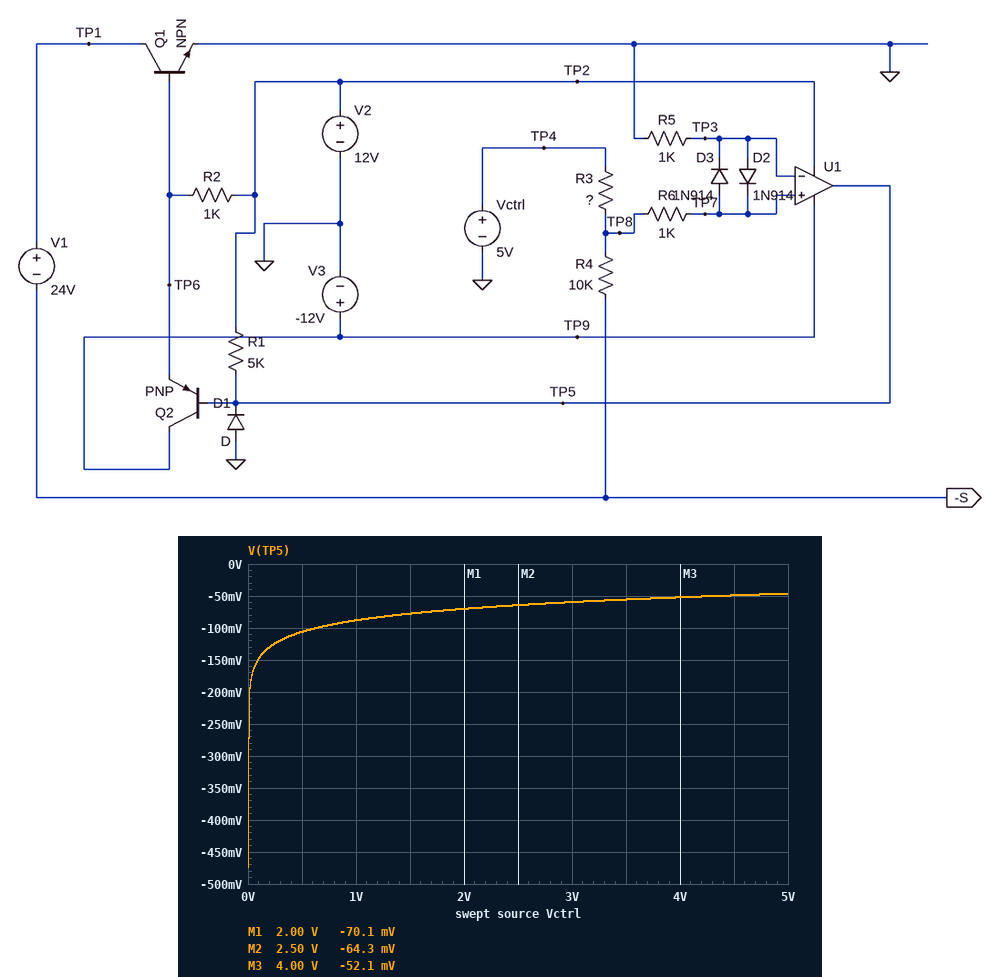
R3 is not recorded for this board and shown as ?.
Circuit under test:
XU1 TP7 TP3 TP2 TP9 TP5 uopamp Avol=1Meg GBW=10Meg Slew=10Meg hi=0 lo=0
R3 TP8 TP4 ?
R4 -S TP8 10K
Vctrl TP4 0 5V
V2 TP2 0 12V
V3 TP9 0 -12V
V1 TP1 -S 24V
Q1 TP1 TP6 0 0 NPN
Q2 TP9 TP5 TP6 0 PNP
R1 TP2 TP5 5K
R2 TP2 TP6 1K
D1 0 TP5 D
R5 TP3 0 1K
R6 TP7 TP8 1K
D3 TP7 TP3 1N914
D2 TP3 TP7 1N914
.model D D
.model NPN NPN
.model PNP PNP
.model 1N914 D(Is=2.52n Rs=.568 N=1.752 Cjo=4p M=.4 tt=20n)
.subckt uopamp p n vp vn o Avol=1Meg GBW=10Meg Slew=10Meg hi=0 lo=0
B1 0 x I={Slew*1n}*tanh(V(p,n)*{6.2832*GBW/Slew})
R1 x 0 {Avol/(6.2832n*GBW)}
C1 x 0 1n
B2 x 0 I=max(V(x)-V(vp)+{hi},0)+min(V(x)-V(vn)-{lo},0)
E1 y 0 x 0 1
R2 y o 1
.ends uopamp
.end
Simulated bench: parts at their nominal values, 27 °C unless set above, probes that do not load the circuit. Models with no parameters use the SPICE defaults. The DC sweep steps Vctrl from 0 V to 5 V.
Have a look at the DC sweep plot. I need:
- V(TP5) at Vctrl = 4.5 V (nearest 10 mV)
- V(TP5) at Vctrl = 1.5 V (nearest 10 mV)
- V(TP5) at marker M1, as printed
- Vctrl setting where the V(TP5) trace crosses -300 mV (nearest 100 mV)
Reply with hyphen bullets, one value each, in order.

- -50 mV
- -80 mV
- -70.1 mV
- 0 V
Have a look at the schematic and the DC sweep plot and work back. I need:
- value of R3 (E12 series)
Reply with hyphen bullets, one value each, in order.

- 2.7 kΩ
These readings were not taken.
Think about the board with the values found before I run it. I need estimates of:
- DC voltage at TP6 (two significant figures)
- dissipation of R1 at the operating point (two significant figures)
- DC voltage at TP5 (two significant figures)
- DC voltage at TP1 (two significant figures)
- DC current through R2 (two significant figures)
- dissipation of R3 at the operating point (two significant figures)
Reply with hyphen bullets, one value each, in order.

- 790 mV
- 29 mW
- -46 mV
- 5.5 V
- 11 mA
- 9.3 mW
